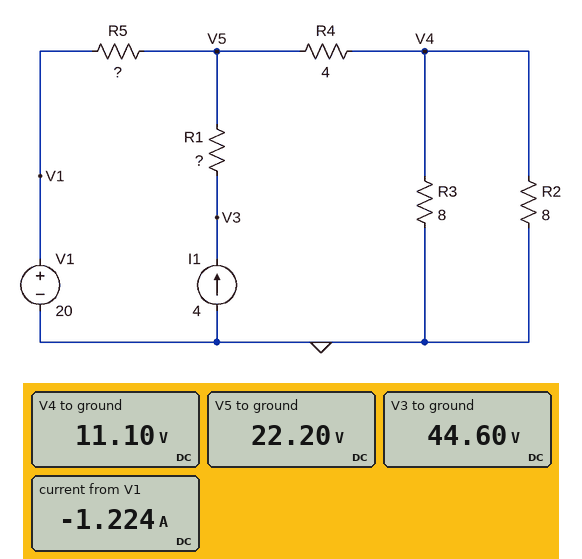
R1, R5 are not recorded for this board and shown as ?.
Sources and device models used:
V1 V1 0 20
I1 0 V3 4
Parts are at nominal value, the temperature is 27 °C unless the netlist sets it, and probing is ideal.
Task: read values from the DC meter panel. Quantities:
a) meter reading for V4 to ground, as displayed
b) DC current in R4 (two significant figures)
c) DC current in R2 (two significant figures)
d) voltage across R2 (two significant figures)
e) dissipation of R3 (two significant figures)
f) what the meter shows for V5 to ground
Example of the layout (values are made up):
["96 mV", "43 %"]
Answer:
["11.10 V", "2.8 A", "1.4 A", "11 V", "15 W", "22.20 V"]
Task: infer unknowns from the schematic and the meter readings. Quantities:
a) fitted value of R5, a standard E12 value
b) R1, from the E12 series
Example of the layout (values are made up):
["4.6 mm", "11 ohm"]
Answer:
["1.8 Ω", "5.6 Ω"]
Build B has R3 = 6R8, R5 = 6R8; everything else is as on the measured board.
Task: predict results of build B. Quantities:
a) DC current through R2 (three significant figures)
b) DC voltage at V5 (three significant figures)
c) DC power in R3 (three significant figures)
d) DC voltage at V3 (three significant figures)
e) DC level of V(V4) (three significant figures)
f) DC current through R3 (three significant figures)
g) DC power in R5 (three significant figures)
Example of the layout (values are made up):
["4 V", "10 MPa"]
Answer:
["1.50 A", "25.0 V", "21.1 W", "47.4 V", "12.0 V", "1.76 A", "3.72 W"]
